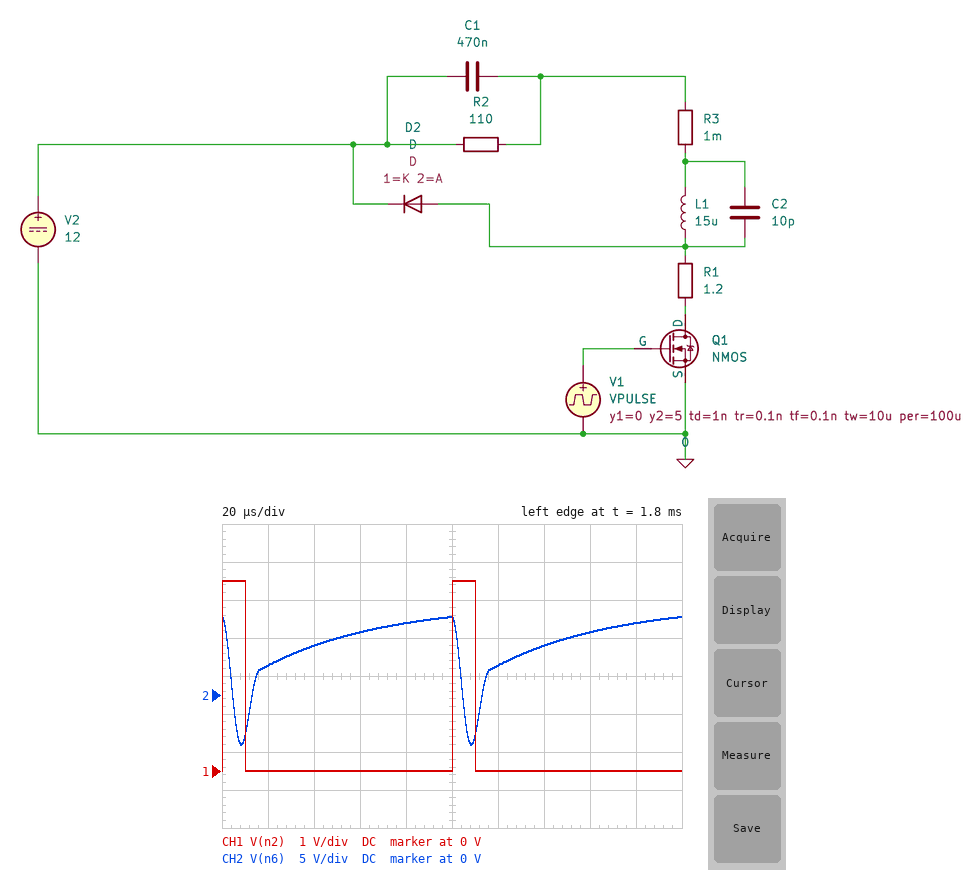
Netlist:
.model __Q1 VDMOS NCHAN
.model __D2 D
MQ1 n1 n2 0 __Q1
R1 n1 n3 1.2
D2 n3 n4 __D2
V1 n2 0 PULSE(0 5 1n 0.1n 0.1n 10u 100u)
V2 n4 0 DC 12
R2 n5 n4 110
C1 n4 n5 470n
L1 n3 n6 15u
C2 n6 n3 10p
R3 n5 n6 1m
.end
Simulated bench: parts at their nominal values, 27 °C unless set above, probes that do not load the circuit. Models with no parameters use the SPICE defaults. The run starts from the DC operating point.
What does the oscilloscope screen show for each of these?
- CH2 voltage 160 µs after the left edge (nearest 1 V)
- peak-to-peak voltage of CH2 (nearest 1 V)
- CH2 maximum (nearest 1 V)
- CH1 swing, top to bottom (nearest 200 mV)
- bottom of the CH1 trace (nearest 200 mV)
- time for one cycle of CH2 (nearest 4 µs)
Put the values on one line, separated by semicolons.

8 V; 17 V; 10 V; 5.0 V; 0 V; 100 µs
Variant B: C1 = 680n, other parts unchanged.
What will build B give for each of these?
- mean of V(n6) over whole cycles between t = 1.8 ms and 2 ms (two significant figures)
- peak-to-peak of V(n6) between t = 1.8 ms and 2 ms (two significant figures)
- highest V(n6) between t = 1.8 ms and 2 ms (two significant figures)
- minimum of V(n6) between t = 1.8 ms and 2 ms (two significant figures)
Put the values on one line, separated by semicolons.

4.9 V; 14 V; 8.7 V; -5.2 V
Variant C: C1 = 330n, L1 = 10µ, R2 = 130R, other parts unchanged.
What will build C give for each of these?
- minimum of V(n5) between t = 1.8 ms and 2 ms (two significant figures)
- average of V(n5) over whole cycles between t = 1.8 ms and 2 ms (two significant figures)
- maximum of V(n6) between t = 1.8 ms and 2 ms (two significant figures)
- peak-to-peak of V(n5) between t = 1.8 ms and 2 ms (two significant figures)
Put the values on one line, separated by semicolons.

-7.1 V; 7.9 V; 11 V; 18 V
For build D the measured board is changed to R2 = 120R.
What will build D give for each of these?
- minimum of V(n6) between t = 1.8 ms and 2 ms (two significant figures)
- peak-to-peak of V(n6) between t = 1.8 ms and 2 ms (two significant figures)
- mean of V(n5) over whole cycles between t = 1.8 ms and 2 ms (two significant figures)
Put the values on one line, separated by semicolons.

-6.4 V; 16 V; 6.2 V
